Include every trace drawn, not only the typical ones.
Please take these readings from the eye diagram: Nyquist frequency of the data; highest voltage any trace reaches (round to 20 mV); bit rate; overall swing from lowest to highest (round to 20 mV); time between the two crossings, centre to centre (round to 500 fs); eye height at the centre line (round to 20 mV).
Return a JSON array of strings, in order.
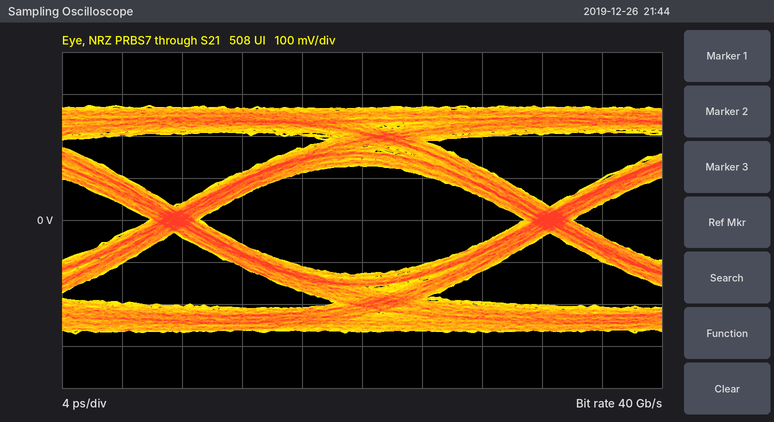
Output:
["20 GHz", "280 mV", "40 Gb/s", "540 mV", "25.0 ps", "260 mV"]
